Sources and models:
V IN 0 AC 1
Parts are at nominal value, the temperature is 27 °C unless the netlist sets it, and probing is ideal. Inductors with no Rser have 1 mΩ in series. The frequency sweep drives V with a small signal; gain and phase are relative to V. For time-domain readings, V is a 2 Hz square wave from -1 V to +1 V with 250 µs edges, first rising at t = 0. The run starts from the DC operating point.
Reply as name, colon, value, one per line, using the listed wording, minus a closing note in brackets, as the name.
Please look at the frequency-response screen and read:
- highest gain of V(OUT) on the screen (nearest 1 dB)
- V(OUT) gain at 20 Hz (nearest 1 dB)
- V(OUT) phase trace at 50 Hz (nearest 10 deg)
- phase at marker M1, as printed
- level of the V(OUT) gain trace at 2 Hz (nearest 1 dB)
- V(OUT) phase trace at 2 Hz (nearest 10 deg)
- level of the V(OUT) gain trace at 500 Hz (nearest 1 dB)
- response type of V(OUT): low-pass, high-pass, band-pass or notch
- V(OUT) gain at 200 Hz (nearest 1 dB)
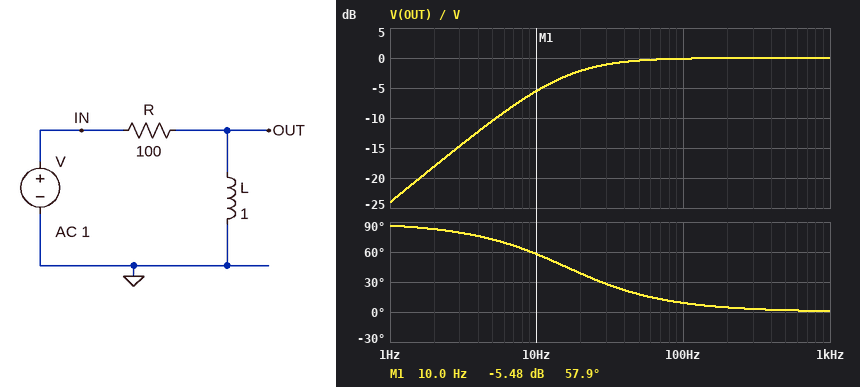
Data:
highest gain of V(OUT) on the screen: 0 dB
V(OUT) gain at 20 Hz: -2 dB
V(OUT) phase trace at 50 Hz: 20 deg
phase at marker M1, as printed: 57.9 deg
level of the V(OUT) gain trace at 2 Hz: -18 dB
V(OUT) phase trace at 2 Hz: 80 deg
level of the V(OUT) gain trace at 500 Hz: 0 dB
response type of V(OUT): low-pass, high-pass, band-pass or notch: high-pass
V(OUT) gain at 200 Hz: 0 dB
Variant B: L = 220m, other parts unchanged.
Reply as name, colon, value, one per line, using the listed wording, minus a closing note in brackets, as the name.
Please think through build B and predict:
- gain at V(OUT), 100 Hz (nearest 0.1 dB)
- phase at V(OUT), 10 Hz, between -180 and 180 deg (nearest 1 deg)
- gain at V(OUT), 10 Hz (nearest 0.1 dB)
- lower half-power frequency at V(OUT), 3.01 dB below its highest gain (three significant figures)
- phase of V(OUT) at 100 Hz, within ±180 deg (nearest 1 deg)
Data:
gain at V(OUT), 100 Hz: -1.8 dB
phase at V(OUT), 10 Hz, between -180 and 180 deg: 82 deg
gain at V(OUT), 10 Hz: -17.3 dB
lower half-power frequency at V(OUT), 3.01 dB below its highest gain: 72.3 Hz
phase of V(OUT) at 100 Hz, within ±180 deg: 36 deg
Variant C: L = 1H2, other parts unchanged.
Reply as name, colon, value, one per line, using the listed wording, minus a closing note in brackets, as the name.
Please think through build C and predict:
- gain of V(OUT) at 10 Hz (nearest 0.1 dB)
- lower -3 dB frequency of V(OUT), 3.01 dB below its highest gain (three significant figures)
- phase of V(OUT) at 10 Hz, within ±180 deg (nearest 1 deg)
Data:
gain of V(OUT) at 10 Hz: -4.4 dB
lower -3 dB frequency of V(OUT), 3.01 dB below its highest gain: 13.3 Hz
phase of V(OUT) at 10 Hz, within ±180 deg: 53 deg
